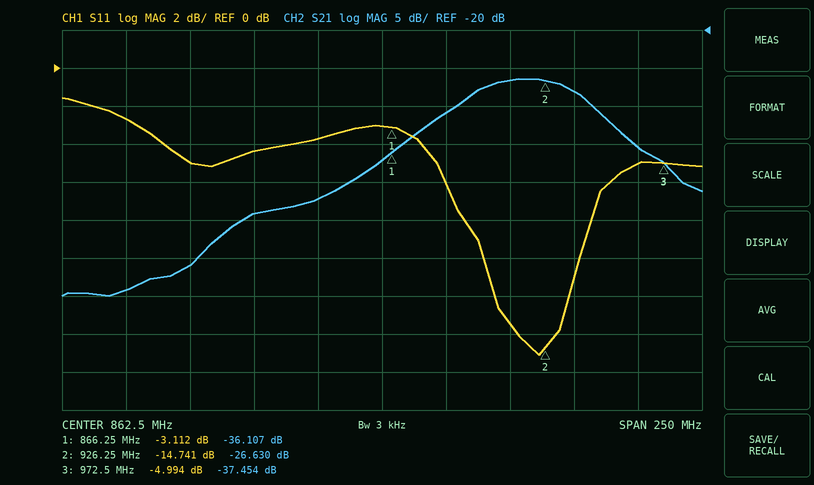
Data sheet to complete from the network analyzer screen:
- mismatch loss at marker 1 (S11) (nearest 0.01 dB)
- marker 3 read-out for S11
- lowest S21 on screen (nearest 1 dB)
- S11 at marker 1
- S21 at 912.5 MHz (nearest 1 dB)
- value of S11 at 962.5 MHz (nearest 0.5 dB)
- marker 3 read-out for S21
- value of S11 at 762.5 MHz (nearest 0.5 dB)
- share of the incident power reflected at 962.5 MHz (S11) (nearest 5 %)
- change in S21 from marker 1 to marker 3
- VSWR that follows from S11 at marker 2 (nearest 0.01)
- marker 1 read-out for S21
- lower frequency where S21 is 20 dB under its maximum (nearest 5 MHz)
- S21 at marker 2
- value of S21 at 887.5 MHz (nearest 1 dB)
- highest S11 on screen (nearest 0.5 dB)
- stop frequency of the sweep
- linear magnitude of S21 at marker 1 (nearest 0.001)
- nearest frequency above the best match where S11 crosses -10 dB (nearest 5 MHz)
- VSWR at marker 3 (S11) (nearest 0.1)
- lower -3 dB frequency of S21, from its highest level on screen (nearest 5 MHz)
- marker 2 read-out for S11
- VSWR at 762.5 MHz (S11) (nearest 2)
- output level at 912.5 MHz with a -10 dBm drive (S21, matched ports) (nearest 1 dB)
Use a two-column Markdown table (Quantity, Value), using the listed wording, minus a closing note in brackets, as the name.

| Quantity | Value |
|---|---|
| mismatch loss at marker 1 (S11) | 2.91 dB |
| marker 3 read-out for S11 | -4.994 dB |
| lowest S21 on screen | -55 dB |
| S11 at marker 1 | -3.112 dB |
| S21 at 912.5 MHz | -27 dB |
| value of S11 at 962.5 MHz | -5.0 dB |
| marker 3 read-out for S21 | -37.454 dB |
| value of S11 at 762.5 MHz | -2.5 dB |
| share of the incident power reflected at 962.5 MHz (S11) | 30 % |
| change in S21 from marker 1 to marker 3 | -1.347 dB |
| VSWR that follows from S11 at marker 2 | 1.45 |
| marker 1 read-out for S21 | -36.107 dB |
| lower frequency where S21 is 20 dB under its maximum | 800 MHz |
| S21 at marker 2 | -26.630 dB |
| value of S21 at 887.5 MHz | -31 dB |
| highest S11 on screen | -1.5 dB |
| stop frequency of the sweep | 987.5 MHz |
| linear magnitude of S21 at marker 1 | 0.016 |
| nearest frequency above the best match where S11 crosses -10 dB | 940 MHz |
| VSWR at marker 3 (S11) | 3.6 |
| lower -3 dB frequency of S21, from its highest level on screen | 895 MHz |
| marker 2 read-out for S11 | -14.741 dB |
| VSWR at 762.5 MHz (S11) | 6 |
| output level at 912.5 MHz with a -10 dBm drive (S21, matched ports) | -37 dBm |
